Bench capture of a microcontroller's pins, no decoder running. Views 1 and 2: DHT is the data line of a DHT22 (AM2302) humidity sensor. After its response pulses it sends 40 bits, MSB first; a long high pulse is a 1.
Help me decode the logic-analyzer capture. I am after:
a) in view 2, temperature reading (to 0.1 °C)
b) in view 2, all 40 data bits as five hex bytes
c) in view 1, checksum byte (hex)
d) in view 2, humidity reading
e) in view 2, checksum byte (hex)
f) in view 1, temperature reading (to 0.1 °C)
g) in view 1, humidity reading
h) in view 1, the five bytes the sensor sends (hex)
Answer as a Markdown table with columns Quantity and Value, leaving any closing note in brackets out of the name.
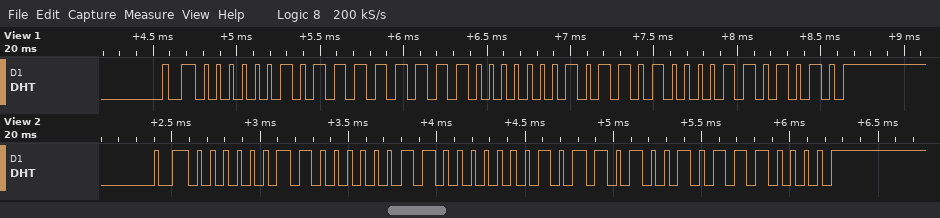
| Quantity | Value |
|---|---|
| in view 2, temperature reading | 36.1 °C |
| in view 2, all 40 data bits as five hex bytes | 03 03 01 69 70 |
| in view 1, checksum byte | 0x6A |
| in view 2, humidity reading | 77.1 % |
| in view 2, checksum byte | 0x70 |
| in view 1, temperature reading | 36.0 °C |
| in view 1, humidity reading | 76.7 % |
| in view 1, the five bytes the sensor sends | 02 FF 01 68 6A |
